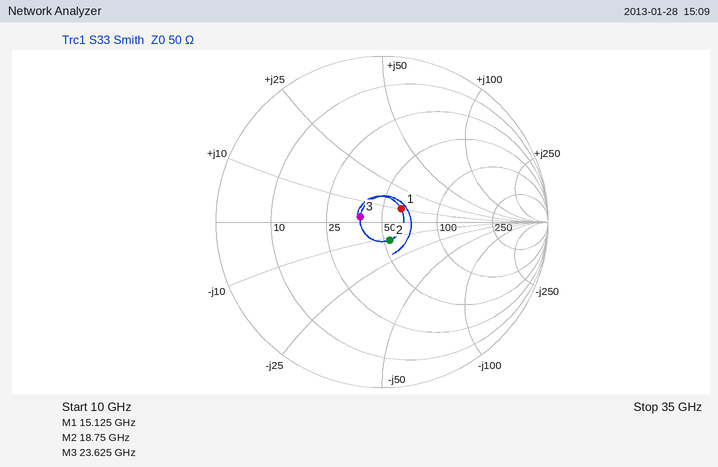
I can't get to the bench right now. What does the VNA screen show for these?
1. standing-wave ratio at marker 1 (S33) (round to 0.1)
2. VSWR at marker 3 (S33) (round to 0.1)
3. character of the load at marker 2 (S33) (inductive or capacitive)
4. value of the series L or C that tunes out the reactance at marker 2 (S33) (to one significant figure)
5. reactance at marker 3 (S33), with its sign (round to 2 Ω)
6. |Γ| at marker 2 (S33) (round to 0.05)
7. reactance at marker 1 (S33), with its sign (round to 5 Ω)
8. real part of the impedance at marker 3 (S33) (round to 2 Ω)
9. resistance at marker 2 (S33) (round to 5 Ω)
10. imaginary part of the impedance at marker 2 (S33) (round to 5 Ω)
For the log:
1.3
1.3
capacitive
100 pH
+2 Ω
0.10
+10 Ω
38 Ω
55 Ω
-10 Ω
